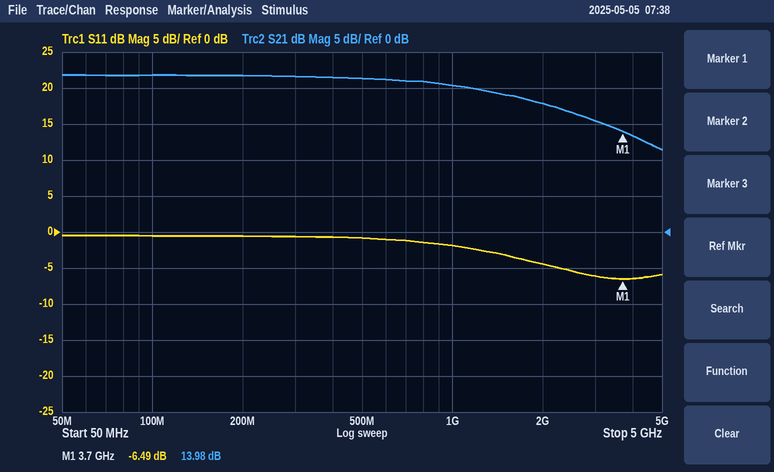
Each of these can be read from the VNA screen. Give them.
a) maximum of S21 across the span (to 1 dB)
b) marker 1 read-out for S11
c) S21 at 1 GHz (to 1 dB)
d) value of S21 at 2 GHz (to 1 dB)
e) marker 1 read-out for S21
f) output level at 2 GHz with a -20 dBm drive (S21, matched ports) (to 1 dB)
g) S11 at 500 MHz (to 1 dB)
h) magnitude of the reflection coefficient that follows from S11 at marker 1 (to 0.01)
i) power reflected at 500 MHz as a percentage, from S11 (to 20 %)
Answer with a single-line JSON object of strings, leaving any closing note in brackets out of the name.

{"maximum of S21 across the span": "22 dB", "marker 1 read-out for S11": "-6.49 dB", "S21 at 1 GHz": "20 dB", "value of S21 at 2 GHz": "18 dB", "marker 1 read-out for S21": "13.98 dB", "output level at 2 GHz with a -20 dBm drive (S21, matched ports)": "-2 dBm", "S11 at 500 MHz": "-1 dB", "magnitude of the reflection coefficient that follows from S11 at marker 1": "0.47", "power reflected at 500 MHz as a percentage, from S11": "80 %"}
